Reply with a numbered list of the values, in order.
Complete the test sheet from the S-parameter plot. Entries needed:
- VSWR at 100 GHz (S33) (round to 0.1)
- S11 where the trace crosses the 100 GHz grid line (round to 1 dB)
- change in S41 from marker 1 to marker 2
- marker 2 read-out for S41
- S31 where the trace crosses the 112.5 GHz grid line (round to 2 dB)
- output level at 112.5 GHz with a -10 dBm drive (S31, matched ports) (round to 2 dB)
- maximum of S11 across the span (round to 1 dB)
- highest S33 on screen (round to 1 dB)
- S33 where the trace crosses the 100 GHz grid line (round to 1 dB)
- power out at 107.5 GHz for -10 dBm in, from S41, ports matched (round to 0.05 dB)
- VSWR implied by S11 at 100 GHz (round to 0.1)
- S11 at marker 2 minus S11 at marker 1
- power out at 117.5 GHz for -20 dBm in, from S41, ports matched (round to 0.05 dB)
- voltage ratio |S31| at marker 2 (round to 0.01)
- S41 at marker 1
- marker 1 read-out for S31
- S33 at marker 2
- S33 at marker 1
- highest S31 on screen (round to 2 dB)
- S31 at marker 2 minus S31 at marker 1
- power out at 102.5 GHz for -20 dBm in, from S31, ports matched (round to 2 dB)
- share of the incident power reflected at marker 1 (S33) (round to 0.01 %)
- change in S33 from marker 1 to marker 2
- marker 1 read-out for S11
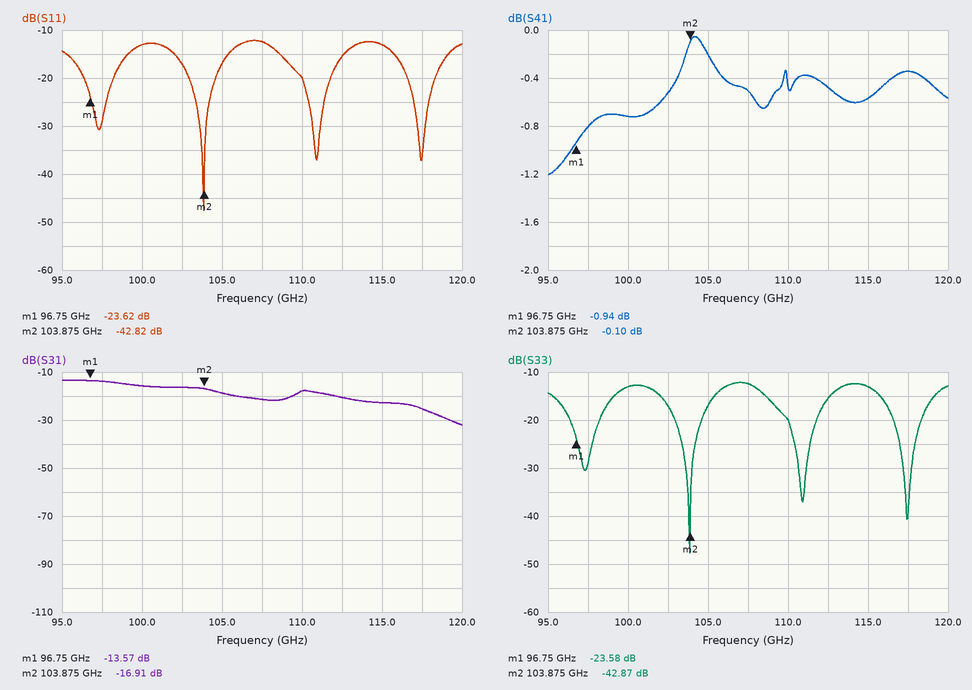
1. 1.6
2. -13 dB
3. 0.84 dB
4. -0.10 dB
5. -20 dB
6. -30 dBm
7. -12 dB
8. -12 dB
9. -13 dB
10. -10.50 dBm
11. 1.6
12. -19.20 dB
13. -20.35 dBm
14. 0.14
15. -0.94 dB
16. -13.57 dB
17. -42.87 dB
18. -23.58 dB
19. -14 dB
20. -3.34 dB
21. -36 dBm
22. 0.44 %
23. -19.29 dB
24. -23.62 dB
